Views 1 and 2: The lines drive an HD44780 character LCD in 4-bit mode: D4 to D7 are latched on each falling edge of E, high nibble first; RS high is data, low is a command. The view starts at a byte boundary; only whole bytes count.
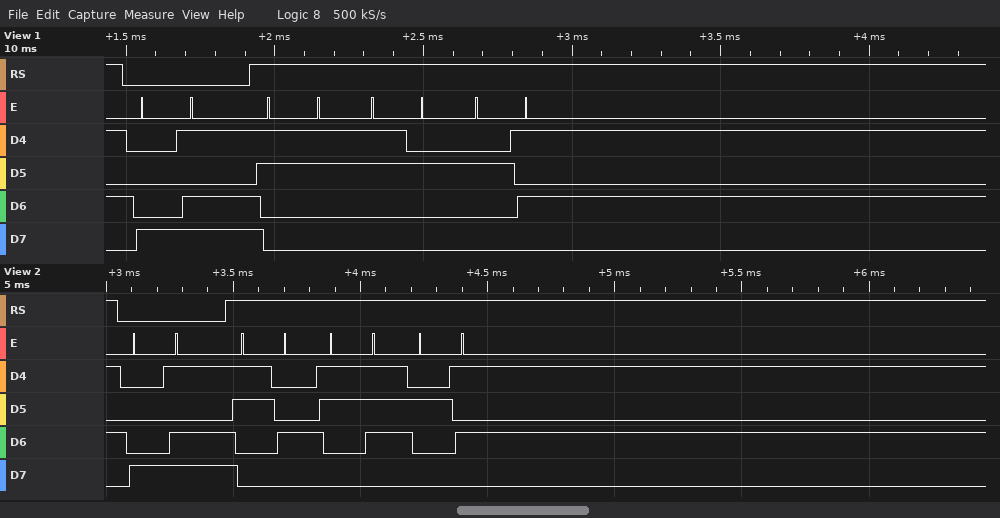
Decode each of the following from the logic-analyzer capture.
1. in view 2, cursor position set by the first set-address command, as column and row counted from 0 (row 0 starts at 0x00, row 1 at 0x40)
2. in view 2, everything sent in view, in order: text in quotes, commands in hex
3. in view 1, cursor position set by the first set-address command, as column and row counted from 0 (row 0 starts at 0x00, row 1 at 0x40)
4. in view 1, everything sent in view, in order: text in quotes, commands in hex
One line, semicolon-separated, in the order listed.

column 13, row 0; 0x8D "47%"; column 13, row 0; 0x8D "32%"
